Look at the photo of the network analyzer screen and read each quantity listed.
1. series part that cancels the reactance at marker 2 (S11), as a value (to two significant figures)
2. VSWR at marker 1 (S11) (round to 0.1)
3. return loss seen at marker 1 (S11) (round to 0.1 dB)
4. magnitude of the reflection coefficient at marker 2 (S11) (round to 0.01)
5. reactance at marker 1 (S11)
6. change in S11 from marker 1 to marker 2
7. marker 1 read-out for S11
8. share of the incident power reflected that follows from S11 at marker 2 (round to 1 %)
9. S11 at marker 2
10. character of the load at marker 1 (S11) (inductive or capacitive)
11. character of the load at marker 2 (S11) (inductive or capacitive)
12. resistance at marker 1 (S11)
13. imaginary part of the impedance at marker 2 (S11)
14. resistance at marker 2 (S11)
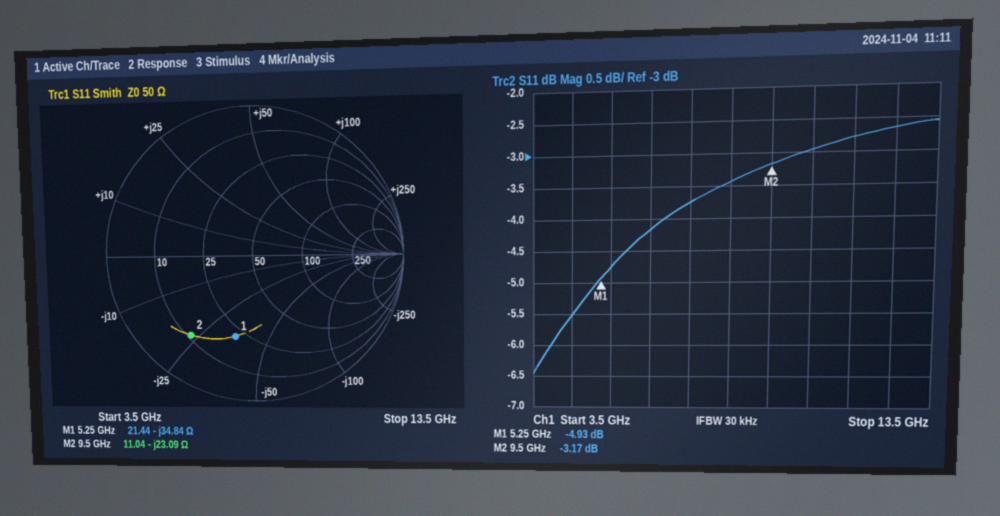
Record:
390 pH
3.6
4.9 dB
0.69
-34.84 Ω
1.76 dB
-4.93 dB
48 %
-3.17 dB
capacitive
capacitive
21.44 Ω
-23.09 Ω
11.04 Ω
